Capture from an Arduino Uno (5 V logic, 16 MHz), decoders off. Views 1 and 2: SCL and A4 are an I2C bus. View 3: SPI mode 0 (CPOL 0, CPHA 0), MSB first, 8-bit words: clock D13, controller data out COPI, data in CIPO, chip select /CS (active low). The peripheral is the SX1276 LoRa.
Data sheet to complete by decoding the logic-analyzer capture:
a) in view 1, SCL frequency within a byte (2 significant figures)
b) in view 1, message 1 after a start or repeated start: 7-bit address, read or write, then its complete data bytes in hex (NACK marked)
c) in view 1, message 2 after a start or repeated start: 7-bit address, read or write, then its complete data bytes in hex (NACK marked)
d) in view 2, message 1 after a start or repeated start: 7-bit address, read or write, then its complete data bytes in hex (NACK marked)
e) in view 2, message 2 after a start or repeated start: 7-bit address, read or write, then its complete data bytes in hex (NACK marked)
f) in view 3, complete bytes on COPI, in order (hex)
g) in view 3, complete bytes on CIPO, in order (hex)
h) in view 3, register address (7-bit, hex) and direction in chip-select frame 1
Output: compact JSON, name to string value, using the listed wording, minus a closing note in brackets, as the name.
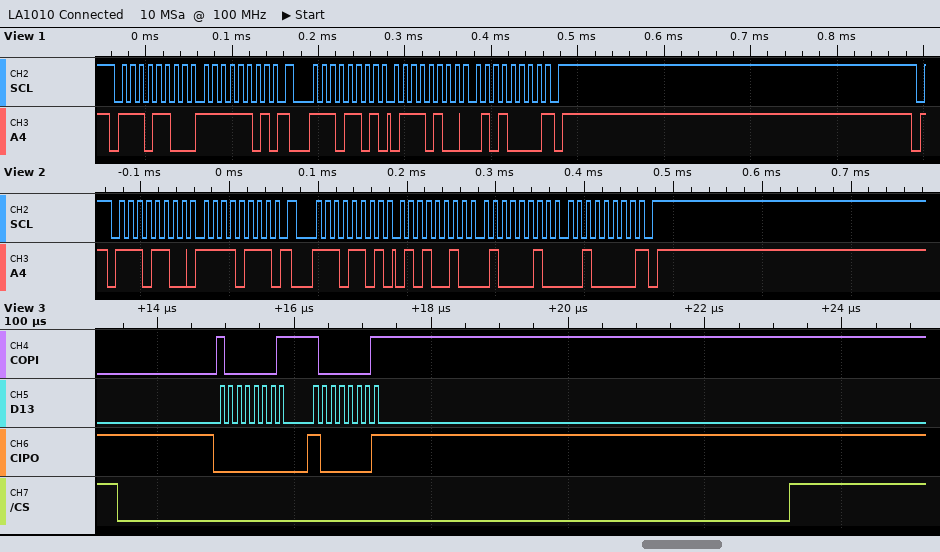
{"in view 1, SCL frequency within a byte": "100 kHz", "in view 1, message 1 after a start or repeated start: 7-bit address, read or write, then its complete data bytes in hex": "0x76 write: FD", "in view 1, message 2 after a start or repeated start: 7-bit address, read or write, then its complete data bytes in hex": "0x76 read: 74 50 NACK", "in view 2, message 1 after a start or repeated start: 7-bit address, read or write, then its complete data bytes in hex": "0x76 write: F7", "in view 2, message 2 after a start or repeated start: 7-bit address, read or write, then its complete data bytes in hex": "0x76 read: 52 42 20 NACK", "in view 3, complete bytes on COPI, in order": "81 81", "in view 3, complete bytes on CIPO, in order": "00 81", "in view 3, register address (7-bit, hex) and direction in chip-select frame 1": "0x01 write"}
